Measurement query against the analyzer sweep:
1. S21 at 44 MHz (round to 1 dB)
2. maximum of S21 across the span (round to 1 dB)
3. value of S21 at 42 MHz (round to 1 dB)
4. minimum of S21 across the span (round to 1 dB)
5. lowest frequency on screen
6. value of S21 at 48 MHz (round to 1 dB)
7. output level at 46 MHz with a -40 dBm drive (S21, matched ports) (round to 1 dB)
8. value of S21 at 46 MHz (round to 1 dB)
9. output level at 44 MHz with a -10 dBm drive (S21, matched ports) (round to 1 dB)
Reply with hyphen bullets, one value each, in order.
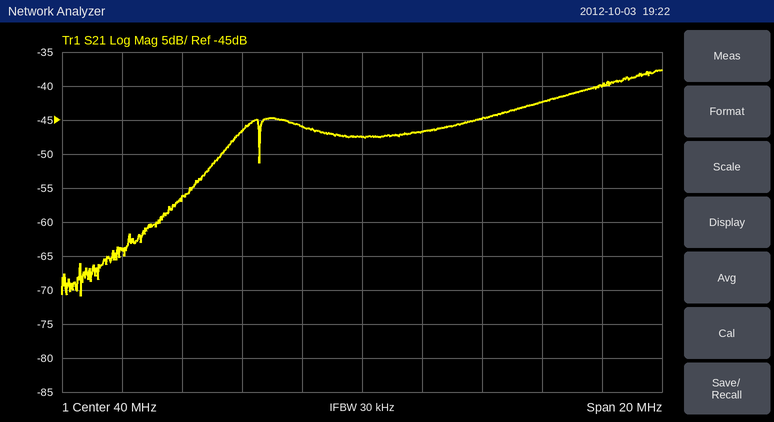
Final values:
- -45 dB
- -38 dB
- -47 dB
- -71 dB
- 30 MHz
- -40 dB
- -82 dBm
- -42 dB
- -55 dBm
